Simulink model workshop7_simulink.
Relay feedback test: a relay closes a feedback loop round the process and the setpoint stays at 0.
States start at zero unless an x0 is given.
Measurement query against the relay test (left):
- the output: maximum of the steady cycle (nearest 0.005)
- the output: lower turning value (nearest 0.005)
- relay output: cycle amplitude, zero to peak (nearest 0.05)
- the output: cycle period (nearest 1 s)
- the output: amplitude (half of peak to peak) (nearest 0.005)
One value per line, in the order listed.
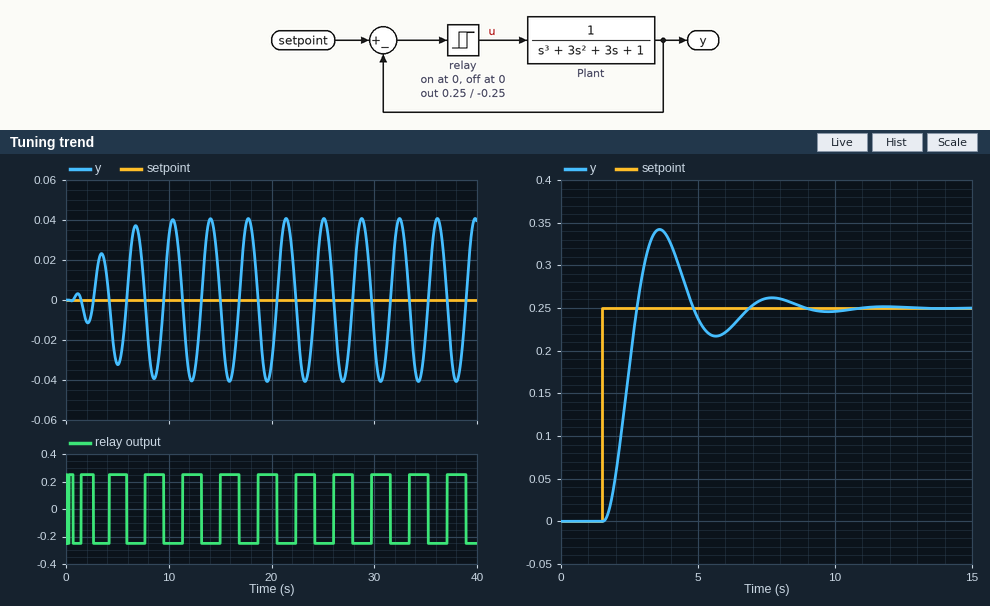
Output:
0.040
-0.040
0.25
4 s
0.040
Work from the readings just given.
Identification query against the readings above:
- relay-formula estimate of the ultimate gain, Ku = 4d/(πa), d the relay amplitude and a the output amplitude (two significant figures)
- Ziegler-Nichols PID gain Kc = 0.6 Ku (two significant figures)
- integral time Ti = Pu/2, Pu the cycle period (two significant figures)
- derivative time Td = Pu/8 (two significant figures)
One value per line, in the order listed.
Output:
8.0
4.8
2.0 s
0.50 s
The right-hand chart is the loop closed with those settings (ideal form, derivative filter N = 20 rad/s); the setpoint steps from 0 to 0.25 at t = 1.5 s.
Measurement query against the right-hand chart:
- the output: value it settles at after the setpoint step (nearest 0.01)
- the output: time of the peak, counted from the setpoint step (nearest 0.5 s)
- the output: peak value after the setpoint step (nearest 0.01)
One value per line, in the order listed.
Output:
0.25
2.0 s
0.34
